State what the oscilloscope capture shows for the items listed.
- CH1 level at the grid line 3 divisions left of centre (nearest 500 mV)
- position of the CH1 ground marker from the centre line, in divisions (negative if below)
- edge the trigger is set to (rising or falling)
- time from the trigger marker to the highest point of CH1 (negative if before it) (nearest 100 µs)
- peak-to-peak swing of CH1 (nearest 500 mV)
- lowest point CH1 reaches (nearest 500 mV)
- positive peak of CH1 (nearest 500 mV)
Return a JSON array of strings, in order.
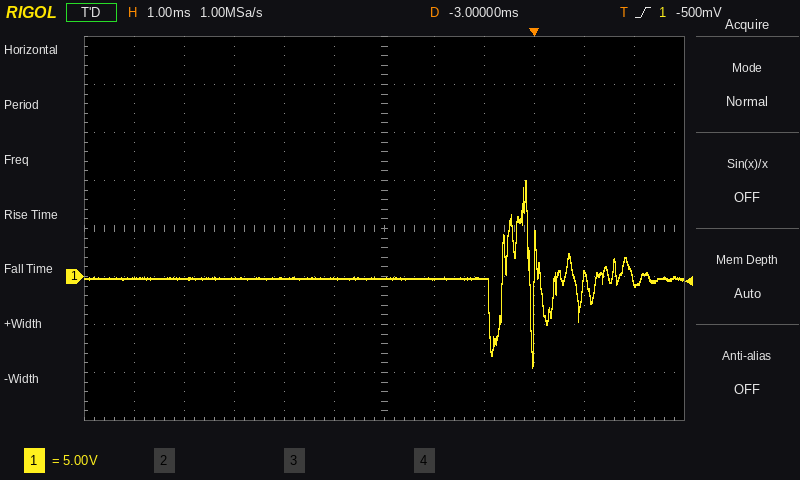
["0.0 V", "-1.0 div", "rising", "-200 µs", "19.5 V", "-9.5 V", "10.0 V"]
